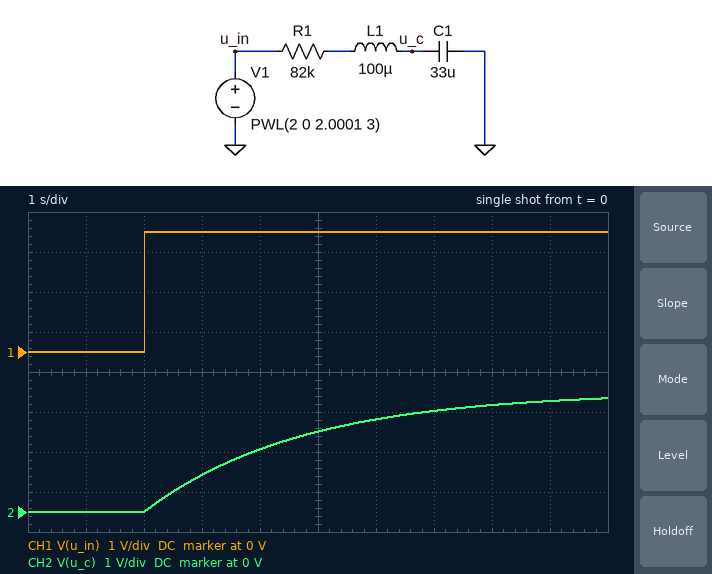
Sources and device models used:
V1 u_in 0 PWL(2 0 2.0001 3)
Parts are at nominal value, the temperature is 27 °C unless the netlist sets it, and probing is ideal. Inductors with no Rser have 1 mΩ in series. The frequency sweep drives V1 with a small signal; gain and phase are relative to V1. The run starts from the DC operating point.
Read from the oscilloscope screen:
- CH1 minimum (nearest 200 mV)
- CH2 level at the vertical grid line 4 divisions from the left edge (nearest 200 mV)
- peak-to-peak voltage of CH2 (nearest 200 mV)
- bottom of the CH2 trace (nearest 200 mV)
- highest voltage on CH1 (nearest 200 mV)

0 V
1.6 V
2.8 V
0 V
3.0 V
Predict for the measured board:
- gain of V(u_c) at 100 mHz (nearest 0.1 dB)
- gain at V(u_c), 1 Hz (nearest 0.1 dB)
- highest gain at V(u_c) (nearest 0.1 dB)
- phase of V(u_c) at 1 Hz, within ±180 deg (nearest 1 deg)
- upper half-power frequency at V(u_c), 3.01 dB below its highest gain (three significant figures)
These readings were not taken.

-5.9 dB
-24.6 dB
0 dB
-87 deg
58.8 mHz
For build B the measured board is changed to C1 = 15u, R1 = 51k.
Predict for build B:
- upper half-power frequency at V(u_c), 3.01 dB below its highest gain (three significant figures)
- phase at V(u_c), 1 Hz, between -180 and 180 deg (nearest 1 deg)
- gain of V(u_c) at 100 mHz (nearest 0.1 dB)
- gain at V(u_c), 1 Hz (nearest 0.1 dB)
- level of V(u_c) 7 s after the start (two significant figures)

208 mHz
-78 deg
-0.9 dB
-13.8 dB
3.0 V
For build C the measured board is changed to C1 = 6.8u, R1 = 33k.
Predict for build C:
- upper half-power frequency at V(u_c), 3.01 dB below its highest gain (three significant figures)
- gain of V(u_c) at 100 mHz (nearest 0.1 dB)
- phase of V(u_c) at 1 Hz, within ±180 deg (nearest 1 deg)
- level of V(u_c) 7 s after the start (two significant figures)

709 mHz
-0.1 dB
-55 deg
3.0 V
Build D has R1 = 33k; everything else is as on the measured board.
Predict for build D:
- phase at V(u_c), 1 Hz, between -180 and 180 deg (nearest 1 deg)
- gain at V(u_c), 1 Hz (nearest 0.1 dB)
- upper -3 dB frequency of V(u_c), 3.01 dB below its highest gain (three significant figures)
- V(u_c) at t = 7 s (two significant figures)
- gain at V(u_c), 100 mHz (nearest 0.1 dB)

-82 deg
-16.8 dB
146 mHz
3.0 V
-1.7 dB
